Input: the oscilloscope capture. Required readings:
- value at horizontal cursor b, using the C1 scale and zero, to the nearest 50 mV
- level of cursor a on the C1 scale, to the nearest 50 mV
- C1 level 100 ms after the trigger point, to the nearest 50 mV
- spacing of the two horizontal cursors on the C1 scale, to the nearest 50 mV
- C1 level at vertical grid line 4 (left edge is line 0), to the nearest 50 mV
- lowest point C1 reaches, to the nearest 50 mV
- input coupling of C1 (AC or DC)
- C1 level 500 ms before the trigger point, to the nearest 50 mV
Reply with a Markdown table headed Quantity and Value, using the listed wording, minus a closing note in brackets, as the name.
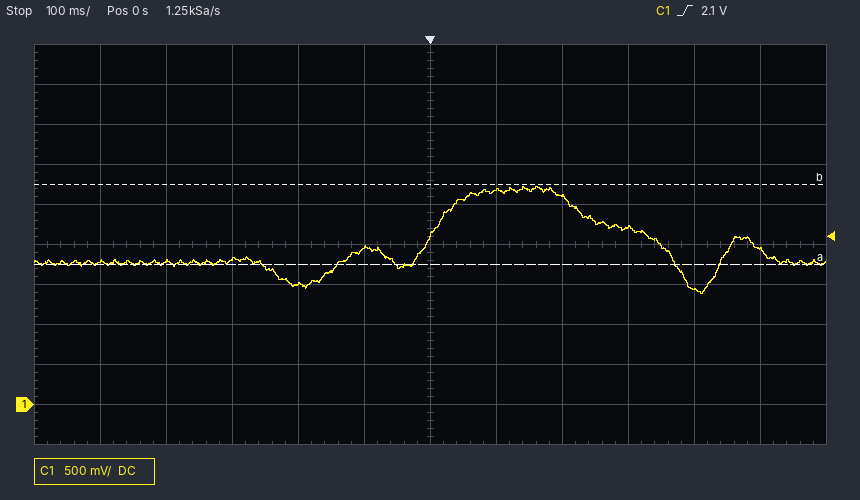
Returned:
| Quantity | Value |
|---|---|
| value at horizontal cursor b, using the C1 scale and zero, to the nearest 50 mV | 2.75 V |
| level of cursor a on the C1 scale, to the nearest 50 mV | 1.75 V |
| C1 level 100 ms after the trigger point, to the nearest 50 mV | 2.70 V |
| spacing of the two horizontal cursors on the C1 scale, to the nearest 50 mV | 1.00 V |
| C1 level at vertical grid line 4 (left edge is line 0), to the nearest 50 mV | 1.50 V |
| lowest point C1 reaches, to the nearest 50 mV | 1.40 V |
| input coupling of C1 | DC |
| C1 level 500 ms before the trigger point, to the nearest 50 mV | 1.80 V |
